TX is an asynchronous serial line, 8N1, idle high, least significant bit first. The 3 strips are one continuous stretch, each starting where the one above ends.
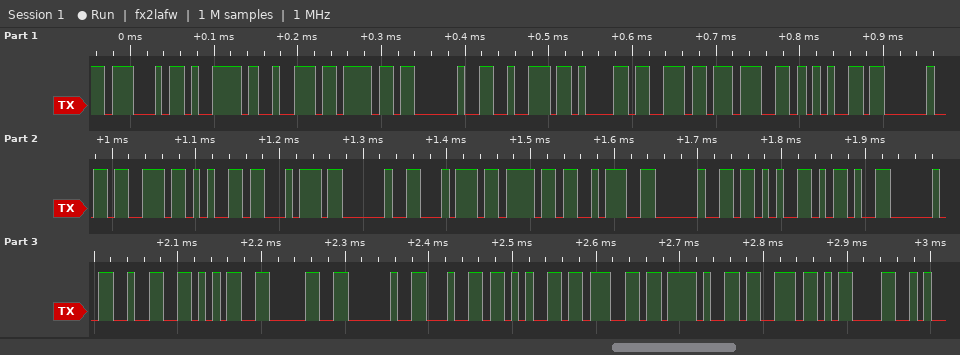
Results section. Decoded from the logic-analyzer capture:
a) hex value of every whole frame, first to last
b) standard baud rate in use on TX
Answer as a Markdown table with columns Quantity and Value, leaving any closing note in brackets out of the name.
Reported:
| Quantity | Value |
|---|---|
| hex value of every whole frame, first to last | 47 79 72 6F 20 72 61 6E 67 65 20 73 65 74 20 74 6F 3A 20 2B 2D 20 32 35 30 20 64 65 67 2F 73 0D |
| standard baud rate in use on TX | 115200 baud |
